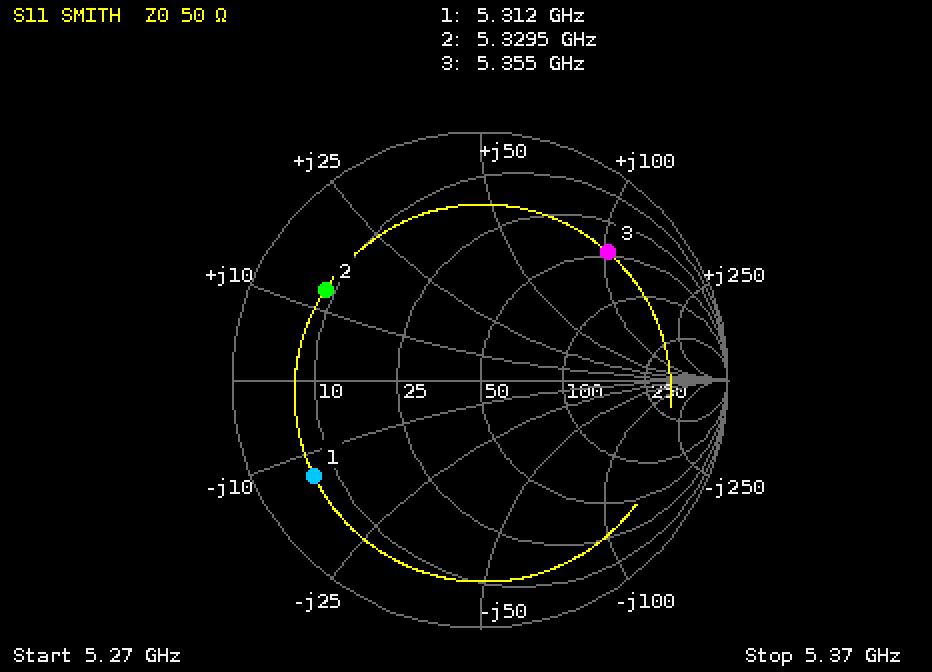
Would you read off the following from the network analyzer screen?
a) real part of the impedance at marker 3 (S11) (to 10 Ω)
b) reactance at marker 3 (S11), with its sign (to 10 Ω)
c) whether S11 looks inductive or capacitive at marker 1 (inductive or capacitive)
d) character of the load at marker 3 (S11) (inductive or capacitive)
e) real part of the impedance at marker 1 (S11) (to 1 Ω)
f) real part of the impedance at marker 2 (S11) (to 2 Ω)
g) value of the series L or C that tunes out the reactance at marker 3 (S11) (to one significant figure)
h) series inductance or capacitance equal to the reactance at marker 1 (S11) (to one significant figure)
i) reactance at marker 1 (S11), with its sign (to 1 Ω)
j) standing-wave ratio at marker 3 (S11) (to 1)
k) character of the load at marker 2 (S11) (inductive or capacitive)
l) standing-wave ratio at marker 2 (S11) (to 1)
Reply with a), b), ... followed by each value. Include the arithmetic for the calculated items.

a) 50 Ω
b) +100 Ω
c) capacitive
d) inductive
e) 7 Ω
f) 8 Ω
g) C = 1/(2π × 5.355 GHz × 100 Ω) ≈ 297 fF, so 300 fF to one significant figure
h) C = 1/(2π × 5.312 GHz × 13 Ω) ≈ 2 pF
i) -13 Ω
j) 6
k) inductive
l) 6
